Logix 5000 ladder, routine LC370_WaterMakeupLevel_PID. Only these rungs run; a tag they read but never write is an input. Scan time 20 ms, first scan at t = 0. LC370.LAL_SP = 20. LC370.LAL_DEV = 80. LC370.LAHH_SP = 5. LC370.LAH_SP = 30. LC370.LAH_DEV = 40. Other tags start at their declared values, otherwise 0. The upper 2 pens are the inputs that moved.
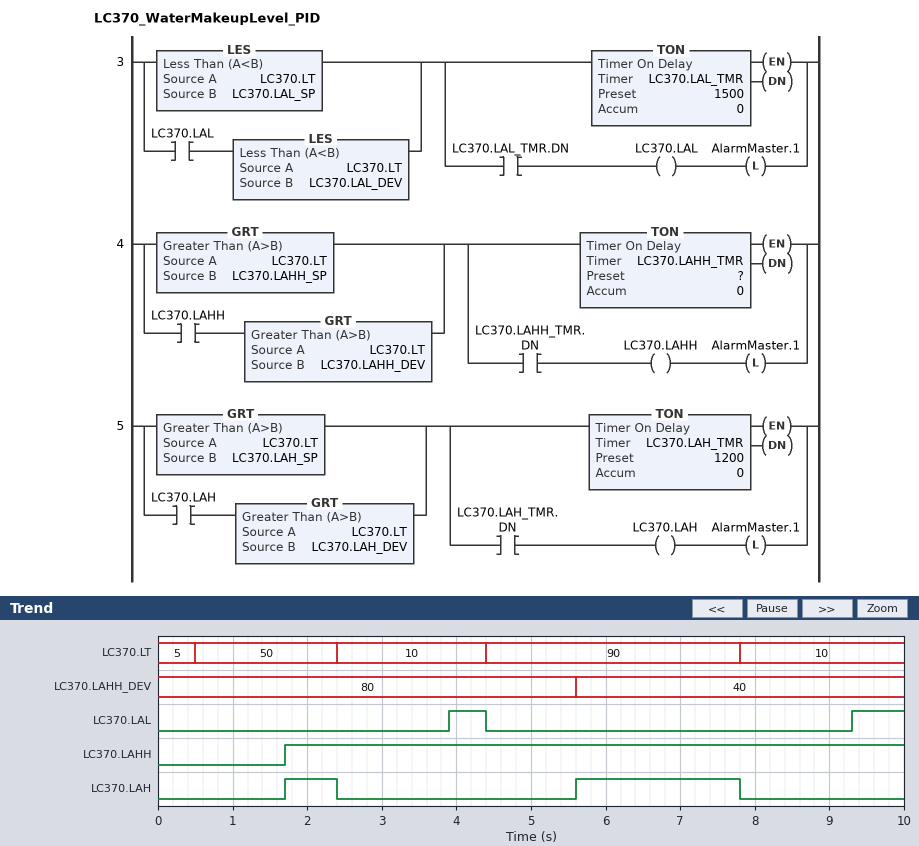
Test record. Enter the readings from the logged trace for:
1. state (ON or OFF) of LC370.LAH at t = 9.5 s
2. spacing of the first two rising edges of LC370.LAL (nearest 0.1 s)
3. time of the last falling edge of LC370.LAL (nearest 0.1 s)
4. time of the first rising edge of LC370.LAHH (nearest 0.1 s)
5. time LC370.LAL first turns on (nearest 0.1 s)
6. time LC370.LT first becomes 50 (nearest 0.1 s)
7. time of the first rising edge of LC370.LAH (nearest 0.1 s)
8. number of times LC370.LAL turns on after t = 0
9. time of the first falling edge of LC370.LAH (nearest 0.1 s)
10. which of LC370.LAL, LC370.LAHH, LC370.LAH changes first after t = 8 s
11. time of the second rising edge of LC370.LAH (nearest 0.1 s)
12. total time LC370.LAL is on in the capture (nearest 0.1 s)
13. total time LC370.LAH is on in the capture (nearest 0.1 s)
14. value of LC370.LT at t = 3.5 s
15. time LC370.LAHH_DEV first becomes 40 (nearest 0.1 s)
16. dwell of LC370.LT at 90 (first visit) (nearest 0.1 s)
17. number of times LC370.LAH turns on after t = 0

OFF
5.4 s
4.4 s
1.7 s
3.9 s
0.5 s
1.7 s
2
2.4 s
LC370.LAL
5.6 s
1.2 s
2.9 s
10
5.6 s
3.4 s
2
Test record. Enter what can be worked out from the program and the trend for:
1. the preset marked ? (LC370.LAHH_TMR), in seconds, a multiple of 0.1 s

1.2 s
